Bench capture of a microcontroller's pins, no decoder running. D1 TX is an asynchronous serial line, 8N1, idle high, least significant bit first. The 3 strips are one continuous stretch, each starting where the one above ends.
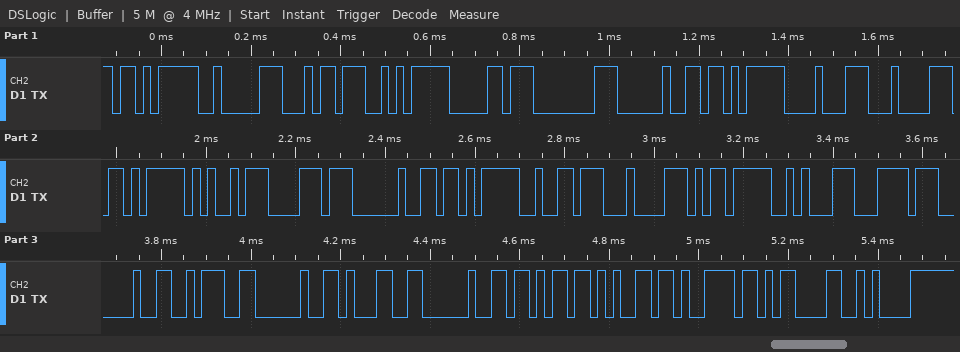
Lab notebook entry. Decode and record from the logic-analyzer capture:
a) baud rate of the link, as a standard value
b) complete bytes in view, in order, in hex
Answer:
57600 baud
EB 82 B4 EA B0 80 20 EB 88 84 EB A5 B8 20 EB B2 84 ED 8A BC 20 3A 20 31 20 6B 65 79 0D 0A
